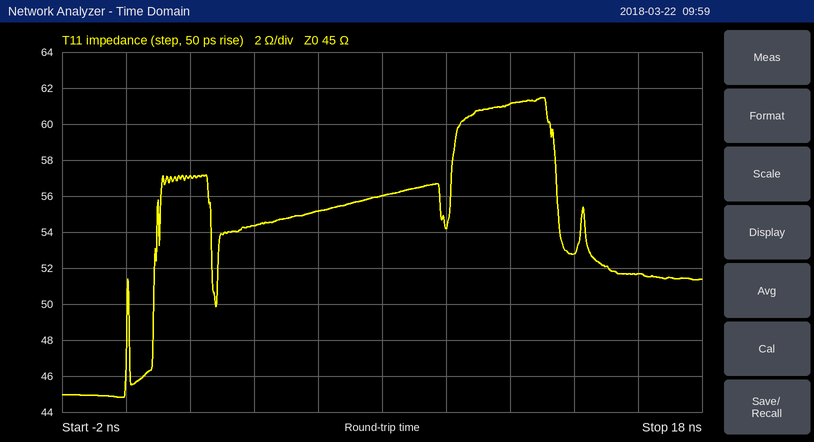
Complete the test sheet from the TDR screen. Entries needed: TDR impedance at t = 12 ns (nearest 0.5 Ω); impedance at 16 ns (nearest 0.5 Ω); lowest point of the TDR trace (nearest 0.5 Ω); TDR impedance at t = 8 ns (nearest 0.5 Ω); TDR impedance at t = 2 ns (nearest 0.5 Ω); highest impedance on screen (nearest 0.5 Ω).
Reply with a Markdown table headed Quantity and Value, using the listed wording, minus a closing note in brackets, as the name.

| Quantity | Value |
|---|---|
| TDR impedance at t = 12 ns | 61.0 Ω |
| impedance at 16 ns | 51.5 Ω |
| lowest point of the TDR trace | 45.0 Ω |
| TDR impedance at t = 8 ns | 56.0 Ω |
| TDR impedance at t = 2 ns | 57.0 Ω |
| highest impedance on screen | 61.5 Ω |
